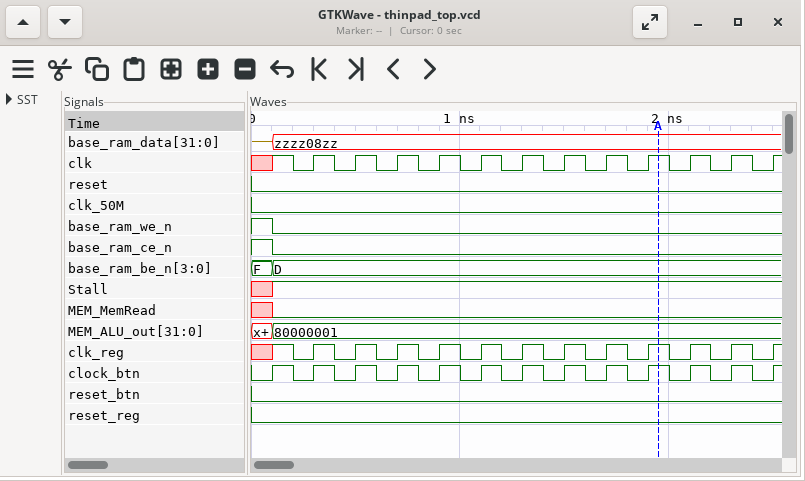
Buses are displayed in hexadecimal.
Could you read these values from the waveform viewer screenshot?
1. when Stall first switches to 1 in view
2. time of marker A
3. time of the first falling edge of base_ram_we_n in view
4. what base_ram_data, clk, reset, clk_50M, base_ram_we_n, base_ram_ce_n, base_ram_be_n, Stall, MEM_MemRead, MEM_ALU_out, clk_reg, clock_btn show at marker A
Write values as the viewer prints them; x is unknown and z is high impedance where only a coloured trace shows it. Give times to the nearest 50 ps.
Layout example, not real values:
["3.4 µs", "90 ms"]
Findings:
["100 ps", "1950 ps", "100 ps", "base_ram_data=zzzz08zz, clk=1, reset=0, clk_50M=0, base_ram_we_n=0, base_ram_ce_n=0, base_ram_be_n=D, Stall=1, MEM_MemRead=0, MEM_ALU_out=80000001, clk_reg=1, clock_btn=1"]
